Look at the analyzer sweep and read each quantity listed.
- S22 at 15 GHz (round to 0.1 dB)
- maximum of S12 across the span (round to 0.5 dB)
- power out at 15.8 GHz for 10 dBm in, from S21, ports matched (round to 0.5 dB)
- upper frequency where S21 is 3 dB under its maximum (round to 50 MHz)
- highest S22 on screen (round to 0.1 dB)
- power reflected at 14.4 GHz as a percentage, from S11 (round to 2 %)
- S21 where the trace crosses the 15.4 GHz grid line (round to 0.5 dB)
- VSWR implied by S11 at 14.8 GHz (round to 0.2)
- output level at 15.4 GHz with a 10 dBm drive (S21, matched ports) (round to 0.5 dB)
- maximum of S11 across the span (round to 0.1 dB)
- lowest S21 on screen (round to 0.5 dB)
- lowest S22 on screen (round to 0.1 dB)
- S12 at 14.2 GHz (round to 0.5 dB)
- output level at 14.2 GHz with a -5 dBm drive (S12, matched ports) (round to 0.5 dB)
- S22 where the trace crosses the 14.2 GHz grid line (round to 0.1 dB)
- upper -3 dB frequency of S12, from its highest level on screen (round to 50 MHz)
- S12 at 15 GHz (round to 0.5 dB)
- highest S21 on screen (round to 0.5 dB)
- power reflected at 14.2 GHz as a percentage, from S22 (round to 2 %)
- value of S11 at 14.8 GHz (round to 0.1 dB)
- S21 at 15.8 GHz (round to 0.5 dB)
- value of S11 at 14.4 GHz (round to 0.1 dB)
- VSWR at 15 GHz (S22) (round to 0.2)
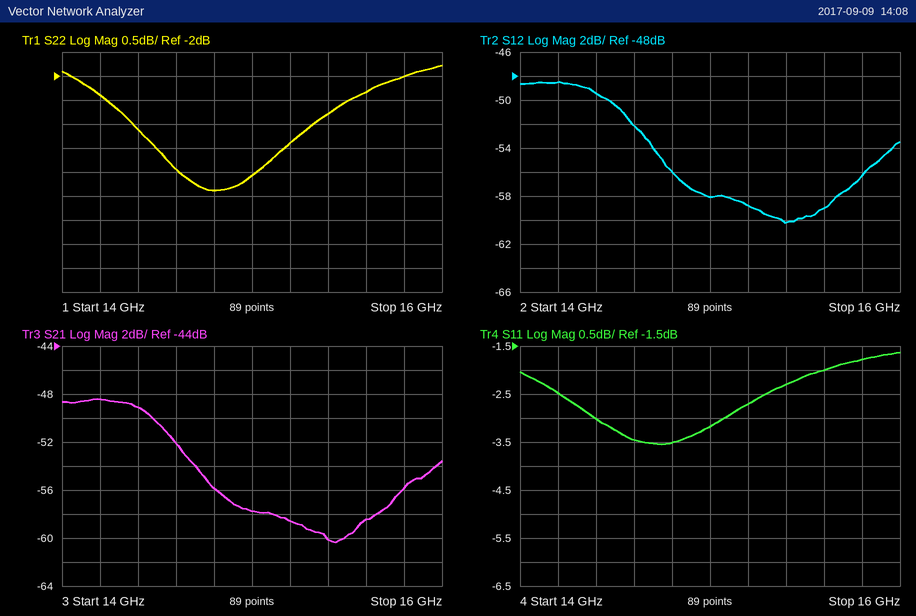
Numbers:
-4.1 dB
-48.5 dB
-46.0 dBm
14.55 GHz
-1.8 dB
50 %
-60.0 dB
5.0
-50.0 dBm
-1.6 dB
-60.5 dB
-4.4 dB
-48.5 dB
-53.5 dBm
-2.4 dB
14.55 GHz
-58.0 dB
-48.5 dB
58 %
-3.5 dB
-56.0 dB
-3.0 dB
4.4
